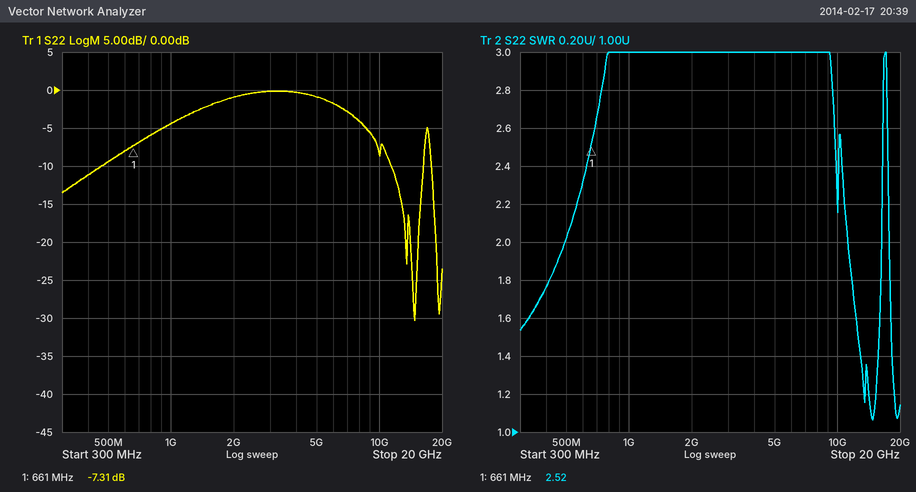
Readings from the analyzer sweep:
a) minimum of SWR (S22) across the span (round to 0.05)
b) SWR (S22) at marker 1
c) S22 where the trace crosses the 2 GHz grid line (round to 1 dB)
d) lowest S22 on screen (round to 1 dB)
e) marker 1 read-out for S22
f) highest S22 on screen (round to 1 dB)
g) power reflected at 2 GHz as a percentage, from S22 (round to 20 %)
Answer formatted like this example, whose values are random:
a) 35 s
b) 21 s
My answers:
a) 1.05
b) 2.52
c) -1 dB
d) -30 dB
e) -7.31 dB
f) 0 dB
g) 80 %
